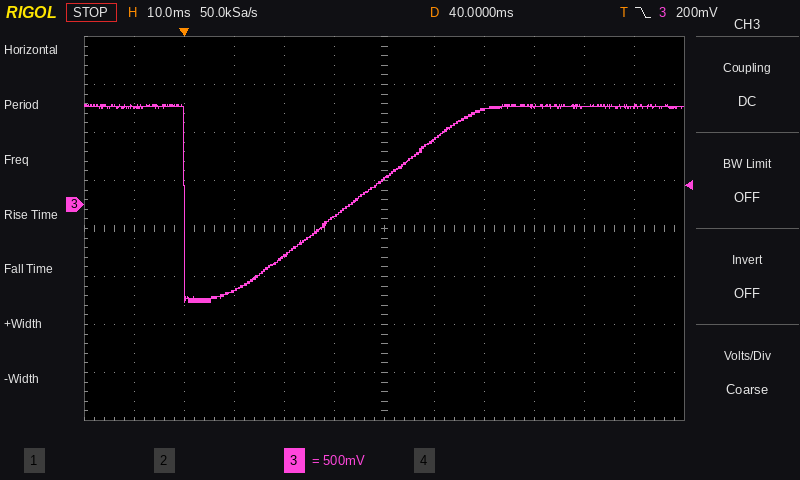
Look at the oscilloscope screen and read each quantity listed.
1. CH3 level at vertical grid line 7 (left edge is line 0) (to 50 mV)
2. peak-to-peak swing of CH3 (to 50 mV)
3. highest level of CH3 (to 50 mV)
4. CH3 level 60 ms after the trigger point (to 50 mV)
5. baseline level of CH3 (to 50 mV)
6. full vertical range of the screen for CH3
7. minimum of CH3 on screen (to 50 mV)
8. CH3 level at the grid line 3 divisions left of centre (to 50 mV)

650 mV
2.05 V
1.05 V
1.00 V
1.00 V
4 V
-1.00 V
-900 mV
